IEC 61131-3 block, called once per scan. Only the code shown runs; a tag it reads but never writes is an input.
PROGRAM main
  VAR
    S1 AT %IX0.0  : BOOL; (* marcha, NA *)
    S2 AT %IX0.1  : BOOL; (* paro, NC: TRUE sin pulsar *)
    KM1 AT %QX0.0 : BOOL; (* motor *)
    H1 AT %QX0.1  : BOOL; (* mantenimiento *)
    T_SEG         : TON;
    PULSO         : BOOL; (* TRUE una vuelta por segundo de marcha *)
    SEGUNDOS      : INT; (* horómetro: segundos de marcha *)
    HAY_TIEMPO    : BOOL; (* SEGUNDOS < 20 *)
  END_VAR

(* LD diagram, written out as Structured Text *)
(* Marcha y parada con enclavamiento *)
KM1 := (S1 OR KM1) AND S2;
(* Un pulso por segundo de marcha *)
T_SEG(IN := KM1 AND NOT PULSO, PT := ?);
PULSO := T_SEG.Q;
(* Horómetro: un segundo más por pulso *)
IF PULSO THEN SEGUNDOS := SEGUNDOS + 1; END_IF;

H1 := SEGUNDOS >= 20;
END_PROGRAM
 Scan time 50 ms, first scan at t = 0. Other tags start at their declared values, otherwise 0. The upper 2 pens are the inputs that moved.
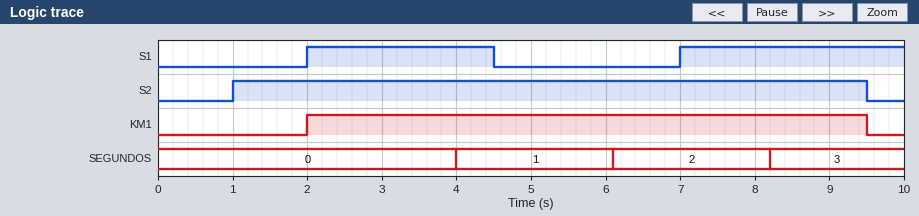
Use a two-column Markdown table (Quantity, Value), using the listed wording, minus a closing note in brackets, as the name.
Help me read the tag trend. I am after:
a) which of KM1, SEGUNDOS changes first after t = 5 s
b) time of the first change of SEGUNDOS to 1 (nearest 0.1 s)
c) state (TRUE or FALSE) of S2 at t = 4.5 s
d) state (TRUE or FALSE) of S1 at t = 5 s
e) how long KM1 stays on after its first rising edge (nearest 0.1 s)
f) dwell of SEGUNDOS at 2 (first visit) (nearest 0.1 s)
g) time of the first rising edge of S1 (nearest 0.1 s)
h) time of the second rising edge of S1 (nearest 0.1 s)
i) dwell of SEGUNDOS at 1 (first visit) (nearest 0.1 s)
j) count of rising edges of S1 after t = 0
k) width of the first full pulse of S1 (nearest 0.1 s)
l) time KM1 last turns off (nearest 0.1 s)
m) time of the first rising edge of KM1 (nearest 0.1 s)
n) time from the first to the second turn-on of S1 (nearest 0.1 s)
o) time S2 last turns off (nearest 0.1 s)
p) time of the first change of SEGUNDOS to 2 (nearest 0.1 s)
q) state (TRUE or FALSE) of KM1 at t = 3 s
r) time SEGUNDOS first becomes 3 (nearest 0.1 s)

| Quantity | Value |
|---|---|
| which of KM1, SEGUNDOS changes first after t = 5 s | SEGUNDOS |
| time of the first change of SEGUNDOS to 1 | 4.0 s |
| state (TRUE or FALSE) of S2 at t = 4.5 s | TRUE |
| state (TRUE or FALSE) of S1 at t = 5 s | FALSE |
| how long KM1 stays on after its first rising edge | 7.5 s |
| dwell of SEGUNDOS at 2 (first visit) | 2.1 s |
| time of the first rising edge of S1 | 2.0 s |
| time of the second rising edge of S1 | 7.0 s |
| dwell of SEGUNDOS at 1 (first visit) | 2.1 s |
| count of rising edges of S1 after t = 0 | 2 |
| width of the first full pulse of S1 | 2.5 s |
| time KM1 last turns off | 9.5 s |
| time of the first rising edge of KM1 | 2.0 s |
| time from the first to the second turn-on of S1 | 5.0 s |
| time S2 last turns off | 9.5 s |
| time of the first change of SEGUNDOS to 2 | 6.1 s |
| state (TRUE or FALSE) of KM1 at t = 3 s | TRUE |
| time SEGUNDOS first becomes 3 | 8.2 s |
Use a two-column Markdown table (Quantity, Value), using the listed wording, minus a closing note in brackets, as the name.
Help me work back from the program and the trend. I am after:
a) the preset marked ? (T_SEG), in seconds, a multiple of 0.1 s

| Quantity | Value |
|---|---|
| the preset marked ? (T_SEG), in seconds, a multiple of 0.1 s | 2.0 s |
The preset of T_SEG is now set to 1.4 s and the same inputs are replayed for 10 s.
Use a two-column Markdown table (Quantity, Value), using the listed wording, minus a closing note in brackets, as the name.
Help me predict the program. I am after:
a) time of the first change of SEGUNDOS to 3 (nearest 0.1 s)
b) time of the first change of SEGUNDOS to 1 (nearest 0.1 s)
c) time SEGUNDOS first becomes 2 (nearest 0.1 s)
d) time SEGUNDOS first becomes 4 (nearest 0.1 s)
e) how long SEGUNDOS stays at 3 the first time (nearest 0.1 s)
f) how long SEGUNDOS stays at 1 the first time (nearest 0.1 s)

| Quantity | Value |
|---|---|
| time of the first change of SEGUNDOS to 3 | 6.4 s |
| time of the first change of SEGUNDOS to 1 | 3.4 s |
| time SEGUNDOS first becomes 2 | 4.9 s |
| time SEGUNDOS first becomes 4 | 7.9 s |
| how long SEGUNDOS stays at 3 the first time | 1.5 s |
| how long SEGUNDOS stays at 1 the first time | 1.5 s |
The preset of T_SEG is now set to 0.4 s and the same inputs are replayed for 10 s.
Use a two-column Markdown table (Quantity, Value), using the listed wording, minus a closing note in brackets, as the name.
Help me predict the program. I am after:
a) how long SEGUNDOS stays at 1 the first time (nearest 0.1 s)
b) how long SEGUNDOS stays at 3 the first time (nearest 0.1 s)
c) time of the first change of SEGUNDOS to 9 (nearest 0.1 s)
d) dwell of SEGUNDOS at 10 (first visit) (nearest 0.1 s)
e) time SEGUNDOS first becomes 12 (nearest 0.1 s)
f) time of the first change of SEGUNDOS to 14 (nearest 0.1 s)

| Quantity | Value |
|---|---|
| how long SEGUNDOS stays at 1 the first time | 0.5 s |
| how long SEGUNDOS stays at 3 the first time | 0.5 s |
| time of the first change of SEGUNDOS to 9 | 6.4 s |
| dwell of SEGUNDOS at 10 (first visit) | 0.5 s |
| time SEGUNDOS first becomes 12 | 7.9 s |
| time of the first change of SEGUNDOS to 14 | 8.9 s |
